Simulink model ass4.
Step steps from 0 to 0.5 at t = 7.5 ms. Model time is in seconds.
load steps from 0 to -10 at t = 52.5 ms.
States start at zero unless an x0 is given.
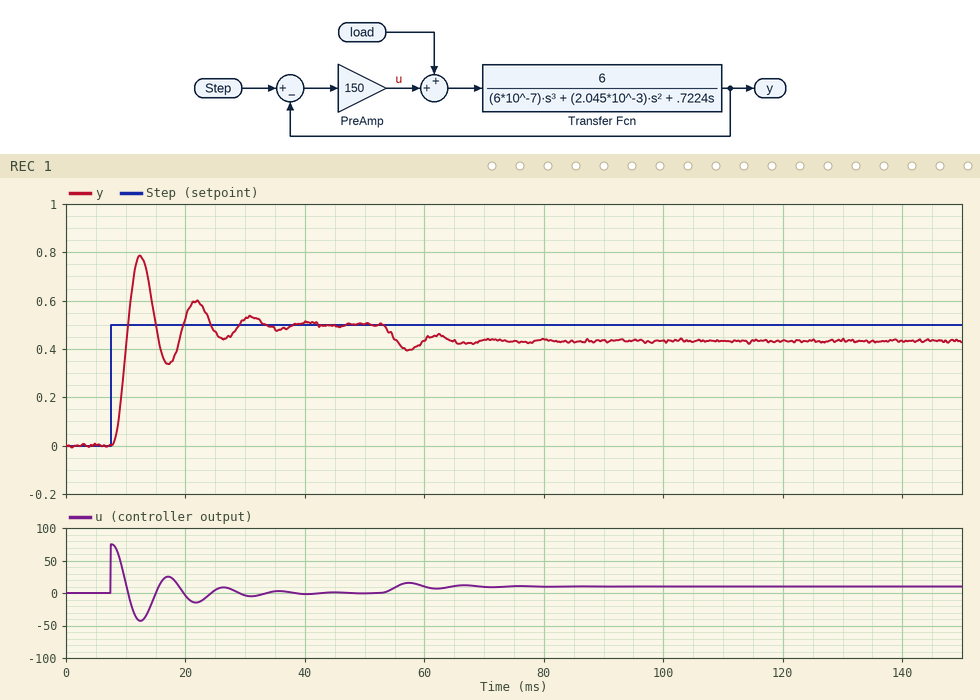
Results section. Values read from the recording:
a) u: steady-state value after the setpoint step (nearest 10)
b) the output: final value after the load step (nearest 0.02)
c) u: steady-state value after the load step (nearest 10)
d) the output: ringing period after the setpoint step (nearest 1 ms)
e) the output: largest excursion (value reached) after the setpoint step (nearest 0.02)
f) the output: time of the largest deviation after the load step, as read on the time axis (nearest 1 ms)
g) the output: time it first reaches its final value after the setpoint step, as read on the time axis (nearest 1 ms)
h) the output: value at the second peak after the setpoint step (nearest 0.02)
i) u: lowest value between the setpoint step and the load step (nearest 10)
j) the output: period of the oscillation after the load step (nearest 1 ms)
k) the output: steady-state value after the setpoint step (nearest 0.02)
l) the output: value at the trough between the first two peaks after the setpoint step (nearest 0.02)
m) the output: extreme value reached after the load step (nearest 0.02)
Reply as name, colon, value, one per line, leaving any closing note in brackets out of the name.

u: steady-state value after the setpoint step: 0
the output: final value after the load step: 0.44
u: steady-state value after the load step: 10
the output: ringing period after the setpoint step: 9 ms
the output: largest excursion (value reached) after the setpoint step: 0.78
the output: time of the largest deviation after the load step, as read on the time axis: 57 ms
the output: time it first reaches its final value after the setpoint step, as read on the time axis: 10 ms
the output: value at the second peak after the setpoint step: 0.60
u: lowest value between the setpoint step and the load step: -40
the output: period of the oscillation after the load step: 9 ms
the output: steady-state value after the setpoint step: 0.50
the output: value at the trough between the first two peaks after the setpoint step: 0.34
the output: extreme value reached after the load step: 0.40
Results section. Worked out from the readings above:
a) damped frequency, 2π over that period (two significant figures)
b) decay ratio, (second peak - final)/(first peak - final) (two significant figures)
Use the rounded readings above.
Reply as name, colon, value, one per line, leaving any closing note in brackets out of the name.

damped frequency, 2π over that period: 0.70 rad/ms
decay ratio, (second peak - final)/(first peak - final): 0.36
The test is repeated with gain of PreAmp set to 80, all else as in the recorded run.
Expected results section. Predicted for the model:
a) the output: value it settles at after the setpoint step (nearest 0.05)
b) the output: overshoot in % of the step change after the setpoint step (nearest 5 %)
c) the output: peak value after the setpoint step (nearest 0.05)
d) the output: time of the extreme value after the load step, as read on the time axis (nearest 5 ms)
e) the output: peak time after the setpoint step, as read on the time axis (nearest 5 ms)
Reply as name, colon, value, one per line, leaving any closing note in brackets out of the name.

the output: value it settles at after the setpoint step: 0.50
the output: overshoot in % of the step change after the setpoint step: 35 %
the output: peak value after the setpoint step: 0.70
the output: time of the extreme value after the load step, as read on the time axis: 60 ms
the output: peak time after the setpoint step, as read on the time axis: 15 ms
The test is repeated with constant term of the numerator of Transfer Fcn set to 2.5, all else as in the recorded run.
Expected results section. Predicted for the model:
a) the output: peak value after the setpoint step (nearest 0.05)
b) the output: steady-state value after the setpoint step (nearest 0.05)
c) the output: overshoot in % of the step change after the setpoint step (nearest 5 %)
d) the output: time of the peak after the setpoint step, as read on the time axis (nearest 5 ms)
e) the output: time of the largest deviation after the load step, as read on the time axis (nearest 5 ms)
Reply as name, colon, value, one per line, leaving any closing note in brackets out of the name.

the output: peak value after the setpoint step: 0.65
the output: steady-state value after the setpoint step: 0.50
the output: overshoot in % of the step change after the setpoint step: 30 %
the output: time of the peak after the setpoint step, as read on the time axis: 15 ms
the output: time of the largest deviation after the load step, as read on the time axis: 60 ms
